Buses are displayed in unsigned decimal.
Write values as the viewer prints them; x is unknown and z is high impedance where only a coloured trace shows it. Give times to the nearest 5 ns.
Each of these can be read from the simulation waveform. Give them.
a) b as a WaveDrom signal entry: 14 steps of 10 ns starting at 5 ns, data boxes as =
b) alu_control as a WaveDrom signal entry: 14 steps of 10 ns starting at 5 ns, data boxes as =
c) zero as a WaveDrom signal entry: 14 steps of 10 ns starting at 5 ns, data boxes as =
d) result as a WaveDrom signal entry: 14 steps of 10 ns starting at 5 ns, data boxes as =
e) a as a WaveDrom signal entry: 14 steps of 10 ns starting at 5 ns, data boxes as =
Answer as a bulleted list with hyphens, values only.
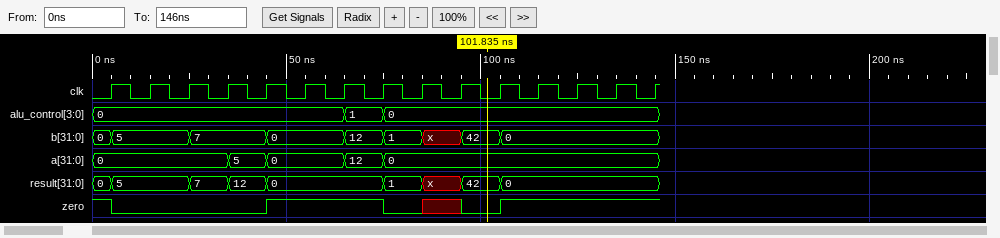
- {name: 'b', wave: '=.=.=.==x==...', data: '5 7 0 12 1 42 0'}
- {name: 'alu_control', wave: '=.....==......', data: '0 1 0'}
- {name: 'zero', wave: '0...1..0x01...'}
- {name: 'result', wave: '=.===..=x==...', data: '5 7 12 0 1 42 0'}
- {name: 'a', wave: '=..==.==......', data: '0 5 0 12 0'}
